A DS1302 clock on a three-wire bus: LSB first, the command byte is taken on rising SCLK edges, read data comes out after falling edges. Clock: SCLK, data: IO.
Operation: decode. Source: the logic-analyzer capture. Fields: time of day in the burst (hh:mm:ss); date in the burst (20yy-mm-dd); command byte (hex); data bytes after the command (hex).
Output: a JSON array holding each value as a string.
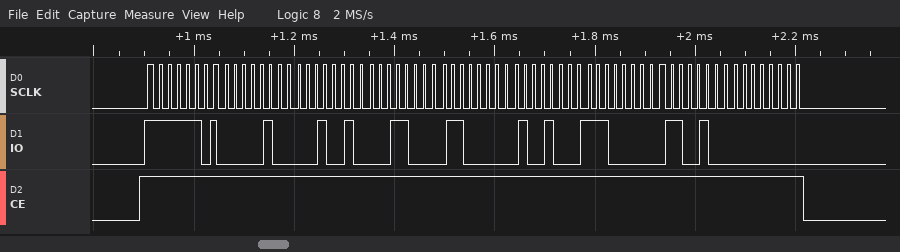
["18:48:20", "2026-12-06", "0xBF", "20 48 18 06 12 07 26 00"]
